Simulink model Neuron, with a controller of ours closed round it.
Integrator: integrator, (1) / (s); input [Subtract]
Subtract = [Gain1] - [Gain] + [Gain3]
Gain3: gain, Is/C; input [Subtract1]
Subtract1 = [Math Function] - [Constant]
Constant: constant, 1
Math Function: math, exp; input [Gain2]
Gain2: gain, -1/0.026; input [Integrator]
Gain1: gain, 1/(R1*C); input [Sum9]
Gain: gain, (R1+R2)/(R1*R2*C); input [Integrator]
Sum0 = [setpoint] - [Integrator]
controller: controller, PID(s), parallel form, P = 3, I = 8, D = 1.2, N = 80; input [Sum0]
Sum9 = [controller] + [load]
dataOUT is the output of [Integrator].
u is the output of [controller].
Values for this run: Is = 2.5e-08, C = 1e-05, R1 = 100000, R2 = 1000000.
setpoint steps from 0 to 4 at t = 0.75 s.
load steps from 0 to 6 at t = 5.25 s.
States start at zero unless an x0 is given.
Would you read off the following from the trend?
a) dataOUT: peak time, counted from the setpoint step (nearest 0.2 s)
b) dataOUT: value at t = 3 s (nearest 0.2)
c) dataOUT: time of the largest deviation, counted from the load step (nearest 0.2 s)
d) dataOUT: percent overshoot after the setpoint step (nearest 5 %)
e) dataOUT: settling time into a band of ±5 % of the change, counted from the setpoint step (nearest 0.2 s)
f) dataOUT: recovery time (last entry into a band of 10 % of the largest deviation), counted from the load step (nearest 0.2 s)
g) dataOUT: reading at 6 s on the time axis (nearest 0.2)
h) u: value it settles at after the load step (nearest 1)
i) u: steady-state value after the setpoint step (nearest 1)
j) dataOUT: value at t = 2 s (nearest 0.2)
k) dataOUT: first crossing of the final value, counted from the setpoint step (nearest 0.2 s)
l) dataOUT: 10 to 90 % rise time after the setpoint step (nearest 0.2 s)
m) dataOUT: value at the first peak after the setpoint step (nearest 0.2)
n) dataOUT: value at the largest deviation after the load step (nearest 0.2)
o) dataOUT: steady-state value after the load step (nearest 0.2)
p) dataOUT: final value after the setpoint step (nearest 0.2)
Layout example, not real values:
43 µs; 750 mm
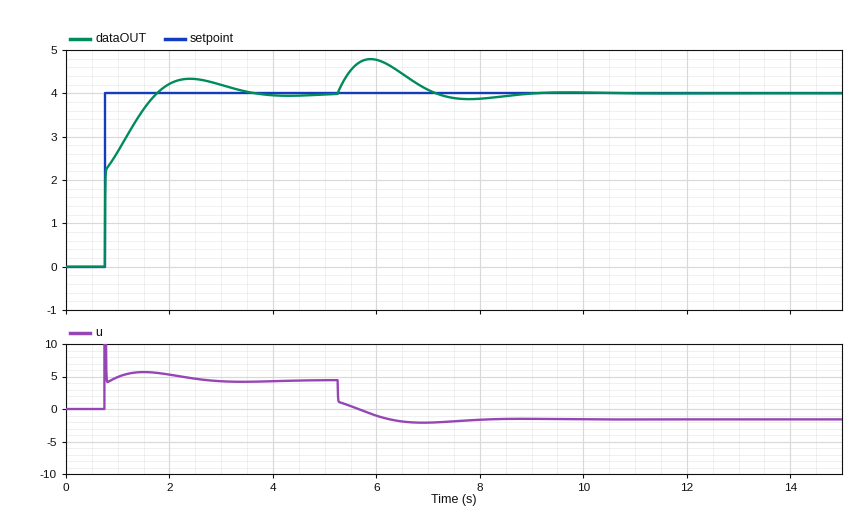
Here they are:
1.6 s; 4.2; 0.6 s; 10 %; 2.2 s; 3.2 s; 4.8; -2; 4; 4.2; 1.0 s; 0.8 s; 4.4; 4.8; 4.0; 4.0
